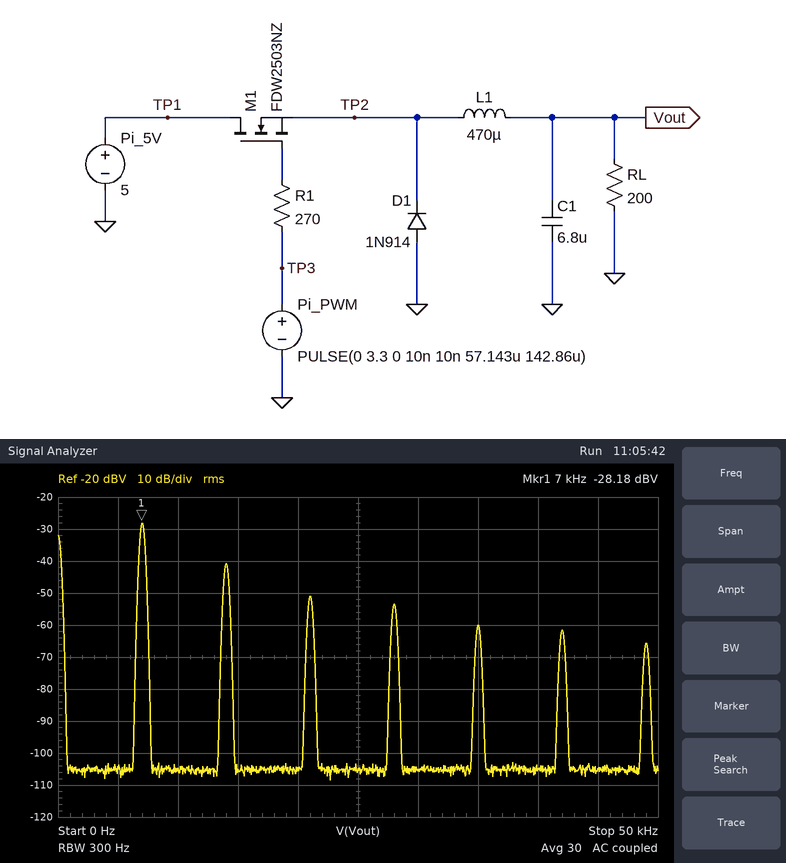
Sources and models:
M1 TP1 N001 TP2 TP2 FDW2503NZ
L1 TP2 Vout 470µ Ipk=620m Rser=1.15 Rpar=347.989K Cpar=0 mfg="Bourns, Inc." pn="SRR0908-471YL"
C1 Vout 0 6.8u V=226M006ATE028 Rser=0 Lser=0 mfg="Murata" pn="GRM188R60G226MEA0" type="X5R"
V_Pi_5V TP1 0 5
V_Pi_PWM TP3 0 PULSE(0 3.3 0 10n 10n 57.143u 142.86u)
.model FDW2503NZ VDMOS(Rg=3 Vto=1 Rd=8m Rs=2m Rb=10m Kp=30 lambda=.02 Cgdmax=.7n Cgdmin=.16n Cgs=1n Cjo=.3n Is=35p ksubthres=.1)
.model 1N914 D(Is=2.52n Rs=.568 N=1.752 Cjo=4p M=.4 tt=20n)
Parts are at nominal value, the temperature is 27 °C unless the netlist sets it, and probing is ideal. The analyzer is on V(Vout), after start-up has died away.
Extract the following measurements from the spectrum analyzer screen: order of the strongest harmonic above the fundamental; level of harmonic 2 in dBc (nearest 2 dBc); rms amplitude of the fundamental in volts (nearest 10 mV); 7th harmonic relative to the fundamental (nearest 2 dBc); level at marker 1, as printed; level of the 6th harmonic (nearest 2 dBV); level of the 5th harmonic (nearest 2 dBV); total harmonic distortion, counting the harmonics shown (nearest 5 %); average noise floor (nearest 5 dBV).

2
-12 dBc
40 mV
-38 dBc
-28.18 dBV
-62 dBV
-60 dBV
25 %
-105 dBV
